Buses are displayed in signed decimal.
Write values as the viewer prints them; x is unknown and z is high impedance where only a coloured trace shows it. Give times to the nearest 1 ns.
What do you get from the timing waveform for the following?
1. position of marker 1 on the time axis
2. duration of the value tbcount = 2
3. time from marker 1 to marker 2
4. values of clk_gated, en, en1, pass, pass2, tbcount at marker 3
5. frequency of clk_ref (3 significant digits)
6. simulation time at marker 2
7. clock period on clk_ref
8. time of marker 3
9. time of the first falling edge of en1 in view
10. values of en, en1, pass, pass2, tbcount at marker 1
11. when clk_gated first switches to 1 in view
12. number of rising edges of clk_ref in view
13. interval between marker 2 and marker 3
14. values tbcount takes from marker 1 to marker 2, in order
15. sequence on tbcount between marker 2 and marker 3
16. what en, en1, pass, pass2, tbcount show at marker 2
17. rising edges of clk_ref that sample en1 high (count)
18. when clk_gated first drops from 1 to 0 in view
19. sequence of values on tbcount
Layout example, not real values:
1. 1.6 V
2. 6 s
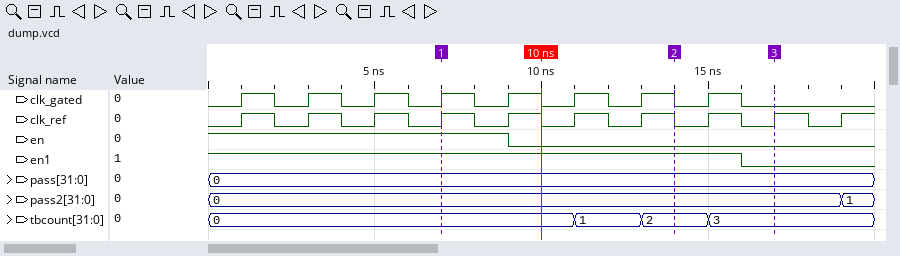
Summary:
1. 7 ns
2. 2 ns
3. 7 ns
4. clk_gated=0, en=0, en1=0, pass=0, pass2=0, tbcount=3
5. 500 MHz
6. 14 ns
7. 2 ns
8. 17 ns
9. 16 ns
10. en=1, en1=1, pass=0, pass2=0, tbcount=0
11. 1 ns
12. 10
13. 3 ns
14. 0, 1, 2
15. 2, 3
16. en=0, en1=1, pass=0, pass2=0, tbcount=2
17. 8
18. 2 ns
19. 0, 1, 2, 3
